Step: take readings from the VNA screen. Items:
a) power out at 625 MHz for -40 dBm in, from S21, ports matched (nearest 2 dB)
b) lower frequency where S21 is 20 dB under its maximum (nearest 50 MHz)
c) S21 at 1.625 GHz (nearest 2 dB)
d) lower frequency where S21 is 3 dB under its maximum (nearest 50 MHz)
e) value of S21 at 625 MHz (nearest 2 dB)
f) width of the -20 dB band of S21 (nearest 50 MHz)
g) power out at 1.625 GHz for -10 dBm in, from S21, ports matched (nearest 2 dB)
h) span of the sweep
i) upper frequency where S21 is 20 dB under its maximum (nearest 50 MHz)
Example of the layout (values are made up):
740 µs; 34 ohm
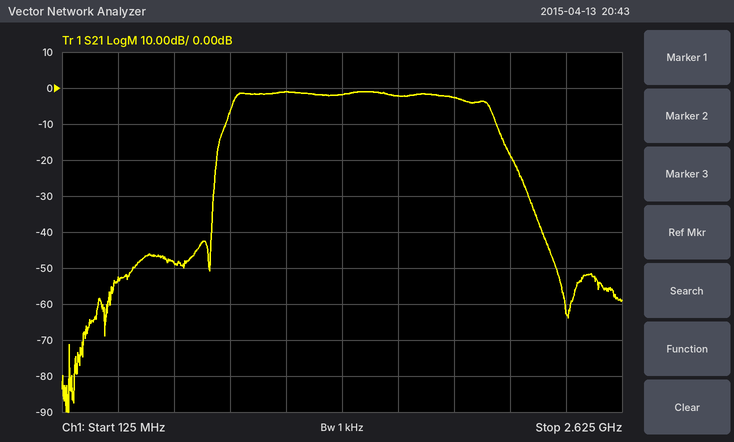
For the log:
-88 dBm; 800 MHz; -2 dB; 900 MHz; -48 dB; 1.35 GHz; -12 dBm; 2.5 GHz; 2.15 GHz
